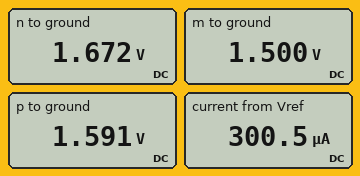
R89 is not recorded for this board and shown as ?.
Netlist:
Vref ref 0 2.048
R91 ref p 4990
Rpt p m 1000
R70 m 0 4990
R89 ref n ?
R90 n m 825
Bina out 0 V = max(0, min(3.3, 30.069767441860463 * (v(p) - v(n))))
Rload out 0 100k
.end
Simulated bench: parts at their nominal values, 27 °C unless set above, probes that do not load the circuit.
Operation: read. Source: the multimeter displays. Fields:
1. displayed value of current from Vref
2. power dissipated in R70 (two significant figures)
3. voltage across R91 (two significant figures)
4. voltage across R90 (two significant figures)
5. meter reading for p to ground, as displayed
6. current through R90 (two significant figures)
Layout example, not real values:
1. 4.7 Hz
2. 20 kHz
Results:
1. 300.5 µA
2. 450 µW
3. 460 mV
4. 170 mV
5. 1.591 V
6. 210 µA
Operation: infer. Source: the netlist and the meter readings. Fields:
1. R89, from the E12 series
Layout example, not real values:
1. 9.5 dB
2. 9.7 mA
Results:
1. 1.8 kΩ
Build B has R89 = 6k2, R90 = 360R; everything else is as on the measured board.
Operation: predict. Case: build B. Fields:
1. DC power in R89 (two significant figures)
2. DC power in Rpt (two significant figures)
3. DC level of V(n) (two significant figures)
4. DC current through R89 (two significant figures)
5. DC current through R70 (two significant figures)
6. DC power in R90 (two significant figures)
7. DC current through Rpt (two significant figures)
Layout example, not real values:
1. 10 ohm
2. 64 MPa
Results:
1. 90 µW
2. 17 µW
3. 1.3 V
4. 120 µA
5. 250 µA
6. 5.2 µW
7. 130 µA
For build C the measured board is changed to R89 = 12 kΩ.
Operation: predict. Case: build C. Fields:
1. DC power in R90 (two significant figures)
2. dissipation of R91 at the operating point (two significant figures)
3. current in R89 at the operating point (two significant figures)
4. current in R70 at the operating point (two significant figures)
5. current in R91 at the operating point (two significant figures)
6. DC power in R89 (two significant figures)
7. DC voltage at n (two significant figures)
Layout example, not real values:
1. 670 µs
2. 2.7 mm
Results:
1. 4.3 µW
2. 120 µW
3. 72 µA
4. 230 µA
5. 150 µA
6. 62 µW
7. 1.2 V
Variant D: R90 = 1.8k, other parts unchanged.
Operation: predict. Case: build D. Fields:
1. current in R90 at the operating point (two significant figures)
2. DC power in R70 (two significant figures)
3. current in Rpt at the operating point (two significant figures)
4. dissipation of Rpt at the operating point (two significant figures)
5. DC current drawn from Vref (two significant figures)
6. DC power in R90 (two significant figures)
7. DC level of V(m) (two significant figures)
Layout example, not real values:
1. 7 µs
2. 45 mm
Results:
1. 180 µA
2. 400 µW
3. 110 µA
4. 11 µW
5. 280 µA
6. 56 µW
7. 1.4 V
